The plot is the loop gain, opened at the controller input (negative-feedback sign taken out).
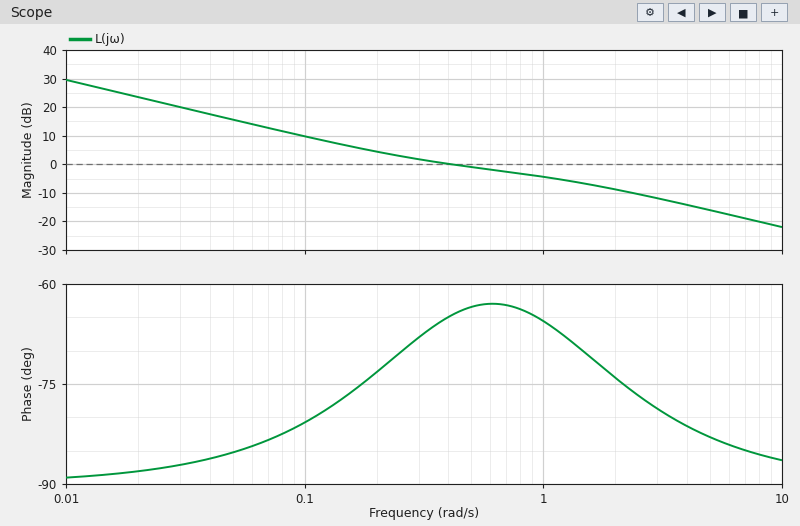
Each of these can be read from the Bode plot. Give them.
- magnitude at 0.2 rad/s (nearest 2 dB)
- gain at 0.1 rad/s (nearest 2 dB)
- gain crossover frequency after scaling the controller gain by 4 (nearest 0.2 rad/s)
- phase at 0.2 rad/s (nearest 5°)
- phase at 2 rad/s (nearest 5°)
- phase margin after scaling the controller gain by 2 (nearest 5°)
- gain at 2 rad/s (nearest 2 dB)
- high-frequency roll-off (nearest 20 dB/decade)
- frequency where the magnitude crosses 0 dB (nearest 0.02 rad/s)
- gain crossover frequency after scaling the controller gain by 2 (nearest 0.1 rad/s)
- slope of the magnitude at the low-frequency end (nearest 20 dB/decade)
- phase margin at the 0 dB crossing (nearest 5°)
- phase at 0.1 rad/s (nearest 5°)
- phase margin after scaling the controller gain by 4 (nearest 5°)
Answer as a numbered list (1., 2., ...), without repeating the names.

1. 4 dB
2. 10 dB
3. 3.0 rad/s
4. -75°
5. -75°
6. 110°
7. -8 dB
8. -20 dB/decade
9. 0.42 rad/s
10. 1.3 rad/s
11. -20 dB/decade
12. 115°
13. -80°
14. 100°
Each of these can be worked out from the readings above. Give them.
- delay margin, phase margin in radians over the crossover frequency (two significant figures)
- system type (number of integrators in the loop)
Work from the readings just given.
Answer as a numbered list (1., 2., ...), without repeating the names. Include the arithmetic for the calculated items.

1. 115 × π / 180 / 0.42 = 4.8 s
2. 1
